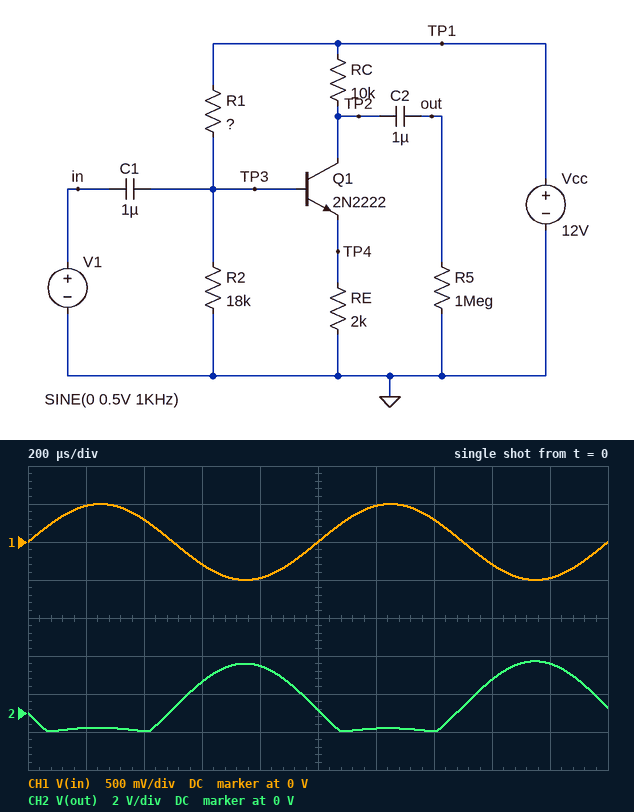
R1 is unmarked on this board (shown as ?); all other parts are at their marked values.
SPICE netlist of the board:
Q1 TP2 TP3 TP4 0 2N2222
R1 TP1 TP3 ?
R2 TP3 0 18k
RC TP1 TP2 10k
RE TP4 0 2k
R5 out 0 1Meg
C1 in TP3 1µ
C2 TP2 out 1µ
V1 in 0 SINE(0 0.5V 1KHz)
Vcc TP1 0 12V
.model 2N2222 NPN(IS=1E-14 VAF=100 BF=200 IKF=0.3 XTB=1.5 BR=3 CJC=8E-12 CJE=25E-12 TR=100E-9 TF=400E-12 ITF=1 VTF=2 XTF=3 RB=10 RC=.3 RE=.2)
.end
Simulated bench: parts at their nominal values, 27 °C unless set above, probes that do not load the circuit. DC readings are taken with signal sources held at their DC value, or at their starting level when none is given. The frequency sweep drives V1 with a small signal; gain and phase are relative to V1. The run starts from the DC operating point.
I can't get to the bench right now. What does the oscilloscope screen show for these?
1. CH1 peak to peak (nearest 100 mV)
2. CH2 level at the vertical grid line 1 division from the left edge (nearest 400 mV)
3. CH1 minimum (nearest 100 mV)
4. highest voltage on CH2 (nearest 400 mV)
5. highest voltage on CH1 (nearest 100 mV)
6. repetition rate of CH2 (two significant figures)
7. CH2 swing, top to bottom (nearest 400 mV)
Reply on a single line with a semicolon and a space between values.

1.0 V; -800 mV; -500 mV; 2.8 V; 500 mV; 1.0 kHz; 3.6 V
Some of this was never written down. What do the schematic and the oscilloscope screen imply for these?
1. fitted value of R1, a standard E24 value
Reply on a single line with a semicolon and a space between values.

68 kΩ
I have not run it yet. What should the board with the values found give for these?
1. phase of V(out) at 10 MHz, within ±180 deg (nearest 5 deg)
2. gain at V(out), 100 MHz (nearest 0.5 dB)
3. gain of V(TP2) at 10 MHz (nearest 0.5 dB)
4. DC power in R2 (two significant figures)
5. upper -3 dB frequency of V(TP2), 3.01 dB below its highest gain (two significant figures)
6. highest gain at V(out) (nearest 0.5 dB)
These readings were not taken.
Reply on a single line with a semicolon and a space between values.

60 deg; 0.5 dB; 4.0 dB; 330 µW; 2.6 MHz; 13.5 dB
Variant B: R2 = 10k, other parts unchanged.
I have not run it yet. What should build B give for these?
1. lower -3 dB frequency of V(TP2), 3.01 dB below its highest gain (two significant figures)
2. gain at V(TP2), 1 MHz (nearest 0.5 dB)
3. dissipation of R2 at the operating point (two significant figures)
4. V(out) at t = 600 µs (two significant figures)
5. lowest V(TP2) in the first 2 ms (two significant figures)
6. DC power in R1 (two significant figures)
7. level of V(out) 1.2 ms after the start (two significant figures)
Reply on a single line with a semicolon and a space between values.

19 Hz; 13.5 dB; 230 µW; 1.5 V; 5.2 V; 1.6 mW; -2.3 V
